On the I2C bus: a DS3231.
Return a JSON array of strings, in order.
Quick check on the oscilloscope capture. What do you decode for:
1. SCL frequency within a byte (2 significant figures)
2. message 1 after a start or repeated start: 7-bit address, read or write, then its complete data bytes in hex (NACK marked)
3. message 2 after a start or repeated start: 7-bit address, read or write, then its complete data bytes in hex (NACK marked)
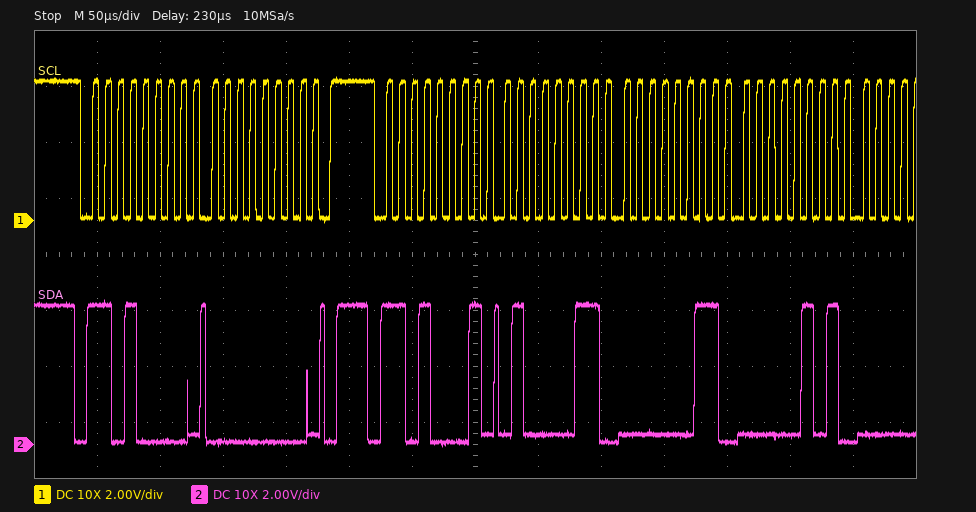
["100 kHz", "0x68 write: 00", "0x68 read: 43 03 05"]
